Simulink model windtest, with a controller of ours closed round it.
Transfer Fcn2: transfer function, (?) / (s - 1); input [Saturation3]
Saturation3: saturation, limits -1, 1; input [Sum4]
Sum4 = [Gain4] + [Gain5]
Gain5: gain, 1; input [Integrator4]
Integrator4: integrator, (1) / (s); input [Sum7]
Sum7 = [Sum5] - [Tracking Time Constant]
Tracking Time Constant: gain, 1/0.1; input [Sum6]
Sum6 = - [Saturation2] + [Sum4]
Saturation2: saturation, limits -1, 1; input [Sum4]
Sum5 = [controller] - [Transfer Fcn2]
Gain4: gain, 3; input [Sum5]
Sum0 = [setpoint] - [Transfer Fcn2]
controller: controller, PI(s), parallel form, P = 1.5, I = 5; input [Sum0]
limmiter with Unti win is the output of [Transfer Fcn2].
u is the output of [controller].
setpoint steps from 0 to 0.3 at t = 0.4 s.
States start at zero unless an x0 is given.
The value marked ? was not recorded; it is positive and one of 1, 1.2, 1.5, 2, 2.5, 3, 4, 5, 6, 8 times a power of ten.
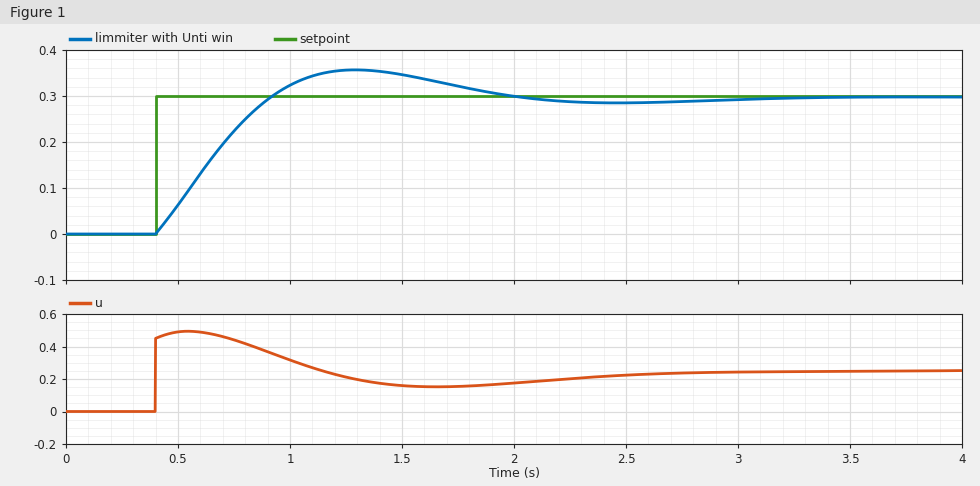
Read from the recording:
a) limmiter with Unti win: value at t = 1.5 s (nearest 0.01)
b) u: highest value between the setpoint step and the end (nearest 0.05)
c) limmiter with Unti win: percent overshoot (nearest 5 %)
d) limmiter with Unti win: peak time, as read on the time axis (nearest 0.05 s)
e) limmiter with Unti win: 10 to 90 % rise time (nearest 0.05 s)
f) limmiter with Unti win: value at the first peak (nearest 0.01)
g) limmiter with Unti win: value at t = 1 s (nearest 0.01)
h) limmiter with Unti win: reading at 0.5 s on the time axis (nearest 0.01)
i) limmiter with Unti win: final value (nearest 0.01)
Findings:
0.35
0.50
20 %
1.30 s
0.40 s
0.36
0.32
0.06
0.30
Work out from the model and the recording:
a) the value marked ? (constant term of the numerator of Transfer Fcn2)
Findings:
0.6
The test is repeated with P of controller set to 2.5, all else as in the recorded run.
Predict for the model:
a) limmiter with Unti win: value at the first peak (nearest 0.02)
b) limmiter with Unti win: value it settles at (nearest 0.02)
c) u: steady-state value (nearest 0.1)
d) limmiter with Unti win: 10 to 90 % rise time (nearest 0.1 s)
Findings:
0.32
0.30
0.3
0.5 s
